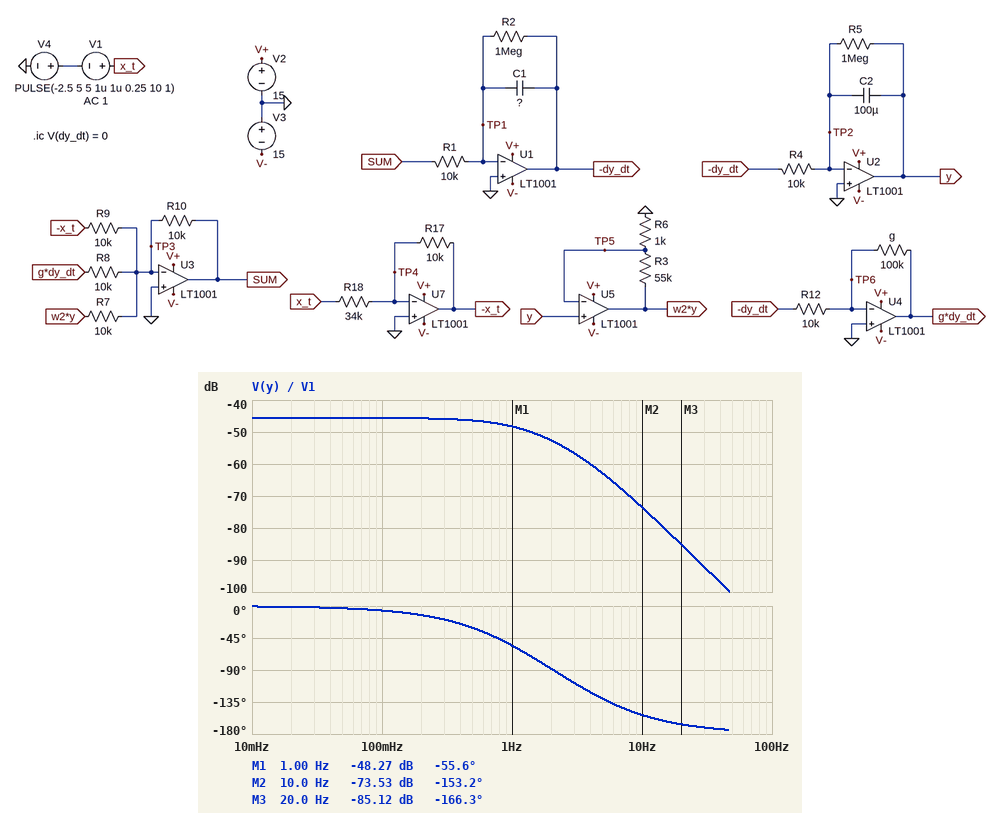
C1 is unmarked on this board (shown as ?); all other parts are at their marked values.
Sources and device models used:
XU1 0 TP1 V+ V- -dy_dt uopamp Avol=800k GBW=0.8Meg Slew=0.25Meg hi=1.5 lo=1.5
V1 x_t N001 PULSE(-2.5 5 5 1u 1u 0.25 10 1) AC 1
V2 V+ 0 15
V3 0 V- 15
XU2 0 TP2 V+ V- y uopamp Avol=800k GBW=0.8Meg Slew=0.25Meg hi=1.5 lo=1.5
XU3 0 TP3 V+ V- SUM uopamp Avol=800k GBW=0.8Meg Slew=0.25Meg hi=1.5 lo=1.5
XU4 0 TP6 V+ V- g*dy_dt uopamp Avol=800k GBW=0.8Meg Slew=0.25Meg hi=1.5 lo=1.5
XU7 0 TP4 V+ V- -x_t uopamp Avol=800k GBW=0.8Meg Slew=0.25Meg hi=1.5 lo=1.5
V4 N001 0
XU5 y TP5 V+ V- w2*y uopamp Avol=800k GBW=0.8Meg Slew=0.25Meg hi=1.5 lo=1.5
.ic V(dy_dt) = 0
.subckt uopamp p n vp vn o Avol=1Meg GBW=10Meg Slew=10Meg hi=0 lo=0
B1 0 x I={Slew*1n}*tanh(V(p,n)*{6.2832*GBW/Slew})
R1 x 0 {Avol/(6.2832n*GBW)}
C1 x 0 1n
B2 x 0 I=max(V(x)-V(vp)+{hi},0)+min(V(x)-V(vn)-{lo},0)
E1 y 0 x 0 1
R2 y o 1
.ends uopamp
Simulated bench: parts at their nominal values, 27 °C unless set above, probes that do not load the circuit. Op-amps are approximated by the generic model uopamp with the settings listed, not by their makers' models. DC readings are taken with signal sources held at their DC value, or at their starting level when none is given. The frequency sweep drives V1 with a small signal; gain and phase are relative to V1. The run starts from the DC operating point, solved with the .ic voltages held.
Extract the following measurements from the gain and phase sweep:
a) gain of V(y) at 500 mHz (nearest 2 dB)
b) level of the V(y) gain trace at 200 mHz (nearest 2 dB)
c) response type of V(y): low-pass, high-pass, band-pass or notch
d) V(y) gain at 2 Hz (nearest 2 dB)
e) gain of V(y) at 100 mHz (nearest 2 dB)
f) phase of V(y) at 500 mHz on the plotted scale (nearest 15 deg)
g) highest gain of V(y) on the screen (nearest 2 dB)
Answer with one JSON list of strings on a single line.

["-46 dB", "-46 dB", "low-pass", "-52 dB", "-46 dB", "-30 deg", "-46 dB"]
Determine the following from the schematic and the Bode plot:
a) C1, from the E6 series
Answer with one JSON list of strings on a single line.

["33 µF"]
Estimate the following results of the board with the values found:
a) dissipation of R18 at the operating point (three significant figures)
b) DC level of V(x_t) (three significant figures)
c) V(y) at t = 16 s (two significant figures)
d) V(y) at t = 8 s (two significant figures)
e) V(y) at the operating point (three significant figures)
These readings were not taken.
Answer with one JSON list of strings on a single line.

["184 µW", "-2.50 V", "-13 mV", "-13 mV", "-13.1 mV"]
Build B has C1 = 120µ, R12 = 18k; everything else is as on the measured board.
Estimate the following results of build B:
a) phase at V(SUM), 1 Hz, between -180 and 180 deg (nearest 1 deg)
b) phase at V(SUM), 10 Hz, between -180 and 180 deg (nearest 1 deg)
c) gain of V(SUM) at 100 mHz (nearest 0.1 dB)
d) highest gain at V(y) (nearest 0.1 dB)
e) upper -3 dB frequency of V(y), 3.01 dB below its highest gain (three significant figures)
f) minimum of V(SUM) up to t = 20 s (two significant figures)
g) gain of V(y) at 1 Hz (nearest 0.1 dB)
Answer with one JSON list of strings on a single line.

["104 deg", "4 deg", "-52.0 dB", "-41.7 dB", "1.29 Hz", "-2.7 V", "-41.8 dB"]
